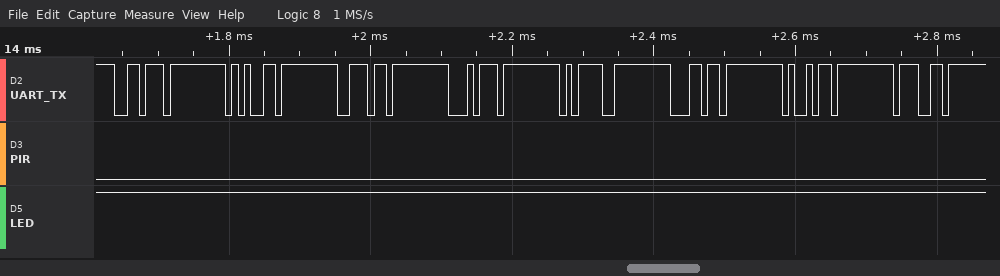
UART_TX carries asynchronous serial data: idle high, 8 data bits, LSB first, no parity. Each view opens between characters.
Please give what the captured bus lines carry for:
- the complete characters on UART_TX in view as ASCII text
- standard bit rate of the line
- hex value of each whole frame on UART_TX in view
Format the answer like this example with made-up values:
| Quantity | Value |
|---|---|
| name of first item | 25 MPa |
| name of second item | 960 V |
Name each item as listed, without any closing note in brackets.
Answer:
| Quantity | Value |
|---|---|
| the complete characters on UART_TX in view as ASCII text | "vent=lig" |
| standard bit rate of the line | 115200 baud |
| hex value of each whole frame on UART_TX in view | 76, 65, 6E, 74, 3D, 6C, 69, 67 |
